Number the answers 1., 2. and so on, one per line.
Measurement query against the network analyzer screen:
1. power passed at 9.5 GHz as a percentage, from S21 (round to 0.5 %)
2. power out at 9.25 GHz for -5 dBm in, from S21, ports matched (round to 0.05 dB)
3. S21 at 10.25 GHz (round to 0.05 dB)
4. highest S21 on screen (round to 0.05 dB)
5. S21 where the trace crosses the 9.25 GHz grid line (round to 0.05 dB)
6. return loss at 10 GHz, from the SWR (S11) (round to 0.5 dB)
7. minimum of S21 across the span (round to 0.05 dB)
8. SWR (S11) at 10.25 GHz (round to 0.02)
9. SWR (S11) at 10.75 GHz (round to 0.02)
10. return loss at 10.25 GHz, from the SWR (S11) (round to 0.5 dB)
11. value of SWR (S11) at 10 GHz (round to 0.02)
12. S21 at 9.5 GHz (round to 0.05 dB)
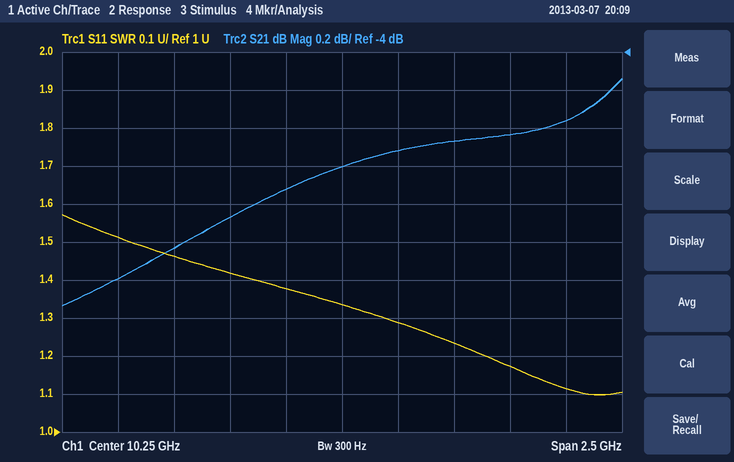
1. 31.5 %
2. -10.20 dBm
3. -4.60 dB
4. -4.15 dB
5. -5.20 dB
6. 16.0 dB
7. -5.35 dB
8. 1.34
9. 1.24
10. 17.0 dB
11. 1.38
12. -5.05 dB
